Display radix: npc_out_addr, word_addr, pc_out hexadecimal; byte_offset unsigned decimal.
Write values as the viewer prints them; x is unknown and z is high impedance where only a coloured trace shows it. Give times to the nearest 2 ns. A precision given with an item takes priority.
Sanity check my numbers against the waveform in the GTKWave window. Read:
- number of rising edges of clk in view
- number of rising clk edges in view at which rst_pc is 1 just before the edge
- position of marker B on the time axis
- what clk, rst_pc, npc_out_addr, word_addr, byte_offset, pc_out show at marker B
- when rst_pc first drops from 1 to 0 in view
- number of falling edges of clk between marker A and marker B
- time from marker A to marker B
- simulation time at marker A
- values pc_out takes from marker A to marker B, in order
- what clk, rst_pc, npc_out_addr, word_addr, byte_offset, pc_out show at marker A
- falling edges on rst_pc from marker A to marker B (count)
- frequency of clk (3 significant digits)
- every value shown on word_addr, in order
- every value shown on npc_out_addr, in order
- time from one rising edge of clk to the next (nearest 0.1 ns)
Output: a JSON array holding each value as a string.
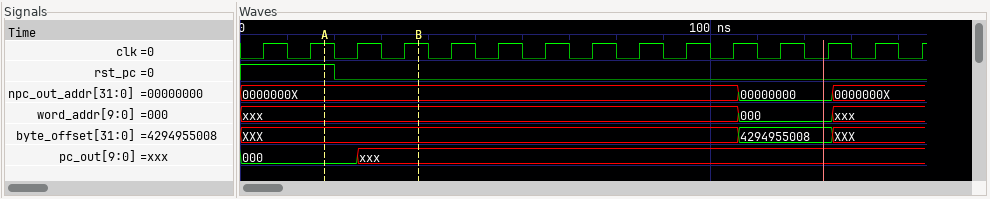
["15", "2", "38 ns", "clk=1, rst_pc=0, npc_out_addr=0000000X, word_addr=xxx, byte_offset=XXX, pc_out=xxx", "20 ns", "2", "20 ns", "18 ns", "000, xxx", "clk=1, rst_pc=1, npc_out_addr=0000000X, word_addr=xxx, byte_offset=XXX, pc_out=000", "1", "100 MHz", "xxx, 000, xxx", "0000000X, 00000000, 0000000X", "10 ns"]
